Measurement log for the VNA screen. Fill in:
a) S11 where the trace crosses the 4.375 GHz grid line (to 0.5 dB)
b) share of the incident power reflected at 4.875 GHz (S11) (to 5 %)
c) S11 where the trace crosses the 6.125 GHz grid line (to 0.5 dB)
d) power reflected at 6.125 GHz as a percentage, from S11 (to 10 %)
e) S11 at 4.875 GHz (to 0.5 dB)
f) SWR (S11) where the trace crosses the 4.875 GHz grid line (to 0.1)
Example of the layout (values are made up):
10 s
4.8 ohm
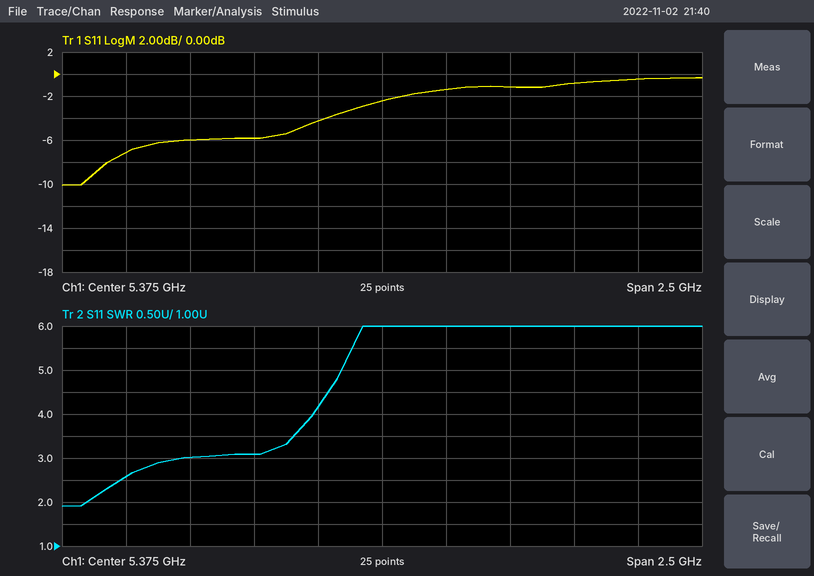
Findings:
-7.0 dB
25 %
-1.0 dB
80 %
-6.0 dB
3.1
